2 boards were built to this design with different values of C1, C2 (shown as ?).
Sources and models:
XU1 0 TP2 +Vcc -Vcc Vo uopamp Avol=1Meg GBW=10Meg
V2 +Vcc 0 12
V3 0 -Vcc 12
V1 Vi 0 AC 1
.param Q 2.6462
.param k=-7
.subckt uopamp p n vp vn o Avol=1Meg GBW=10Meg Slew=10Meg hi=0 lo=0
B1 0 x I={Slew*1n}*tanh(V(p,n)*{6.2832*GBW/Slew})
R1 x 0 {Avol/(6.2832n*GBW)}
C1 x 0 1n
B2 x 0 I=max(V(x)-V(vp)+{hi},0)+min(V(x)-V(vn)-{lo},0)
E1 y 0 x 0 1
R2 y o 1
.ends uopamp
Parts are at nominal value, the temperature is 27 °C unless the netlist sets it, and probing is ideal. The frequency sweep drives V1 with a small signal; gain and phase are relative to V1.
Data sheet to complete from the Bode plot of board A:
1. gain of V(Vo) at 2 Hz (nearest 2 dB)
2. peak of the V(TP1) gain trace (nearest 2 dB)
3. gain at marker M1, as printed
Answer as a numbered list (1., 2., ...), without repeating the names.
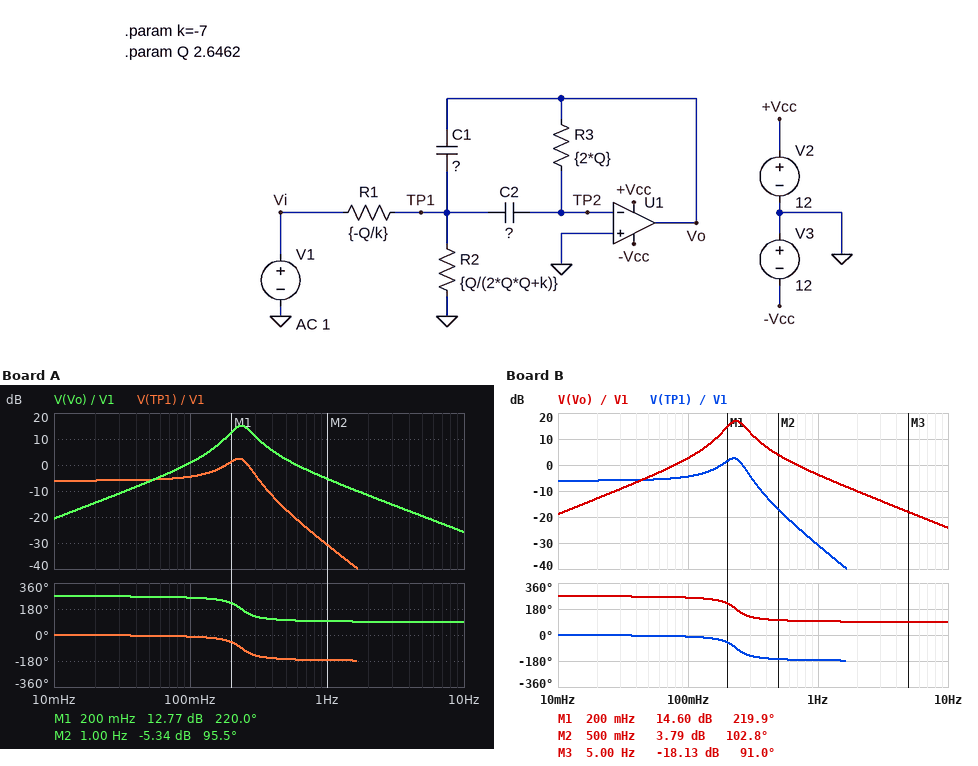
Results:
1. -12 dB
2. 2 dB
3. 12.77 dB
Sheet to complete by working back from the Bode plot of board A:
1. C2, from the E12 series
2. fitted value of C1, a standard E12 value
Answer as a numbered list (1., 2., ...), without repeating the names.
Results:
1. 560 mF
2. 820 mF
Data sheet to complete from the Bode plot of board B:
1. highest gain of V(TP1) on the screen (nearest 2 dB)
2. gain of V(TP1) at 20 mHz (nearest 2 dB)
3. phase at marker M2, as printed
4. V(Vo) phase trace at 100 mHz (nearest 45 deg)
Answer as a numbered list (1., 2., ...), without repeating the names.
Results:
1. 2 dB
2. -6 dB
3. 102.8 deg
4. 270 deg
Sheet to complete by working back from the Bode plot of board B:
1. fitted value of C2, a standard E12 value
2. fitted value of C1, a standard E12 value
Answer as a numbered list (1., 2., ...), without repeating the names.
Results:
1. 680 mF
2. 680 mF
